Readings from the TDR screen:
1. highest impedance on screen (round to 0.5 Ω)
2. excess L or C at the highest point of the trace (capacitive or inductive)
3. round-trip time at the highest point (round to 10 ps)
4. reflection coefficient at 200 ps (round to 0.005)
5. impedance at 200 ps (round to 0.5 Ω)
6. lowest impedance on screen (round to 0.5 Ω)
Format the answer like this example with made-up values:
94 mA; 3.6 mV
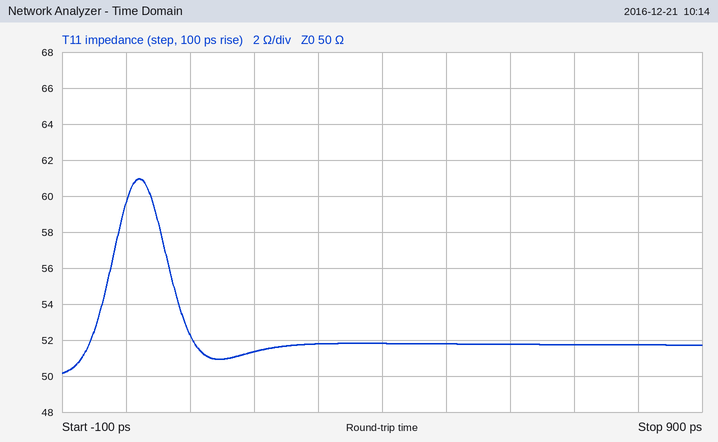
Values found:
61.0 Ω; inductive; 20 ps; +0.015; 51.5 Ω; 50.0 Ω
